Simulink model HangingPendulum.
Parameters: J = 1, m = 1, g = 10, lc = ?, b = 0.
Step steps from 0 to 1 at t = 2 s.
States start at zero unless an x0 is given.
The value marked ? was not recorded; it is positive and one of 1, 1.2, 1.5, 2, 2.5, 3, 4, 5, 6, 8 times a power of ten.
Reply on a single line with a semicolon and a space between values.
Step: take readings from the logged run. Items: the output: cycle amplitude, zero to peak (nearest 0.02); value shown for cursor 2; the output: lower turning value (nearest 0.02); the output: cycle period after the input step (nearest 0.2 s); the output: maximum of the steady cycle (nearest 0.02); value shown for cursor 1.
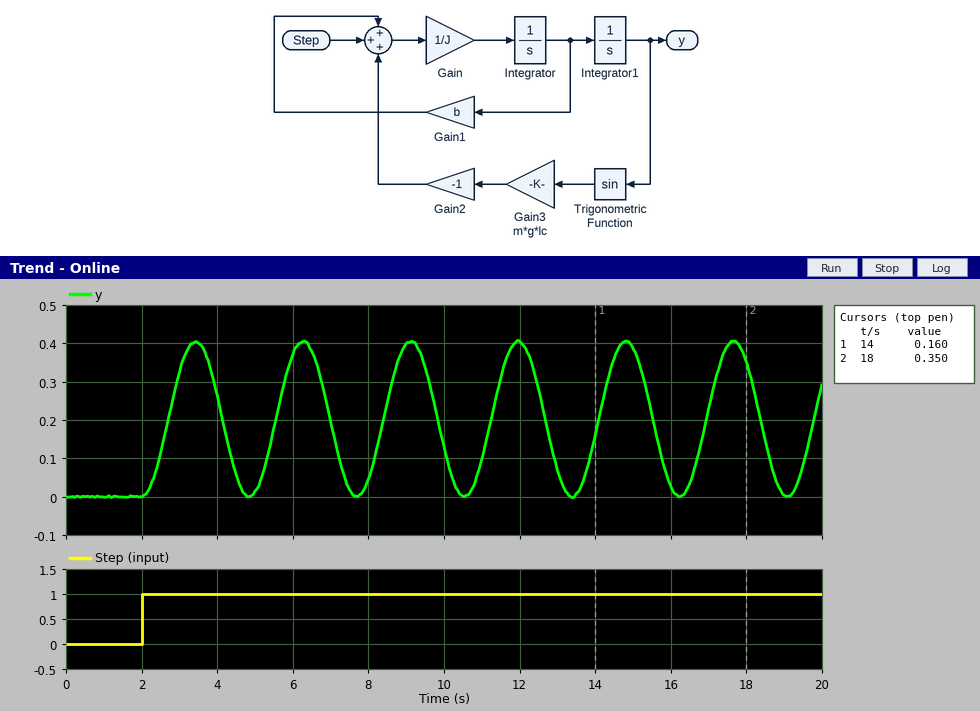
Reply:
0.20; 0.350; 0.00; 2.8 s; 0.40; 0.160
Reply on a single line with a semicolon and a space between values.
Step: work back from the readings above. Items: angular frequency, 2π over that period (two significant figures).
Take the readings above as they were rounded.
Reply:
2.2 rad/s
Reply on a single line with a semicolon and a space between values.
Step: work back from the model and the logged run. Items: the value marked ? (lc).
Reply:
0.5
